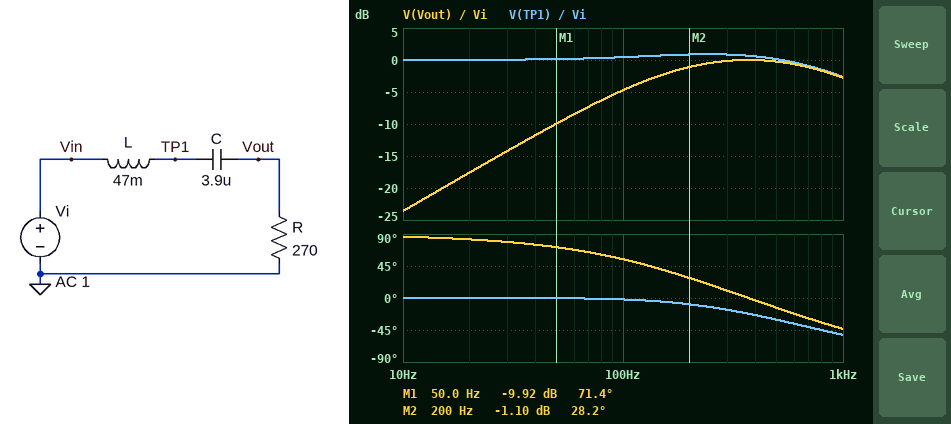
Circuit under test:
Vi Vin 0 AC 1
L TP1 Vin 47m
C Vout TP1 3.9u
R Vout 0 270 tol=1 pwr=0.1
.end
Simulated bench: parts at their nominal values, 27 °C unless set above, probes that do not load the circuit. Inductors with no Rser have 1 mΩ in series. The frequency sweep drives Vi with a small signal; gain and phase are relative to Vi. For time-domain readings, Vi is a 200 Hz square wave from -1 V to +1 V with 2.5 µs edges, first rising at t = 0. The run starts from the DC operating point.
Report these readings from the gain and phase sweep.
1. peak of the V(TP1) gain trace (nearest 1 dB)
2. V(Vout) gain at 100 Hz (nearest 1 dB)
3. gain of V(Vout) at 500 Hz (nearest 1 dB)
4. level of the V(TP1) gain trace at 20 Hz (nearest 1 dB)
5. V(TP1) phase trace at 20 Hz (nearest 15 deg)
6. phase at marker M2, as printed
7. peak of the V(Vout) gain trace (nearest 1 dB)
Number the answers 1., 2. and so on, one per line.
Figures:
1. 1 dB
2. -5 dB
3. 0 dB
4. 0 dB
5. 0 deg
6. 28.2 deg
7. 0 dB
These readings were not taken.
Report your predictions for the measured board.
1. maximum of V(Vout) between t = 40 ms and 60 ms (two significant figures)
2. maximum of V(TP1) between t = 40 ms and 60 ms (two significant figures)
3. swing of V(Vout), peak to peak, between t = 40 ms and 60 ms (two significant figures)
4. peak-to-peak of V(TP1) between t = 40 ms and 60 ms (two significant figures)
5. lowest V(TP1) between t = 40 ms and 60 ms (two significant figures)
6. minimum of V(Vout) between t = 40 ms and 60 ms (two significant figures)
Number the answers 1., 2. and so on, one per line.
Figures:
1. 1.5 V
2. 1.2 V
3. 2.9 V
4. 2.4 V
5. -1.2 V
6. -1.5 V
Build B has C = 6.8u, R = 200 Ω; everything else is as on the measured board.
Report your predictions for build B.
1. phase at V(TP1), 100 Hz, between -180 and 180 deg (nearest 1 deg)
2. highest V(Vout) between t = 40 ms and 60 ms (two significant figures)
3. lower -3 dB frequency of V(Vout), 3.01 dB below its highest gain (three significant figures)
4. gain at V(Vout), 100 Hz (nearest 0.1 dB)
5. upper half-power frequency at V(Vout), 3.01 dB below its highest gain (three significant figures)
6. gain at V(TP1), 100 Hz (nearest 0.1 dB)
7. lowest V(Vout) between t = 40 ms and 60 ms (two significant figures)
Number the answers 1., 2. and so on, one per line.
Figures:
1. -4 deg
2. 1.4 V
3. 102 Hz
4. -3.1 dB
5. 779 Hz
6. 0.6 dB
7. -1.4 V
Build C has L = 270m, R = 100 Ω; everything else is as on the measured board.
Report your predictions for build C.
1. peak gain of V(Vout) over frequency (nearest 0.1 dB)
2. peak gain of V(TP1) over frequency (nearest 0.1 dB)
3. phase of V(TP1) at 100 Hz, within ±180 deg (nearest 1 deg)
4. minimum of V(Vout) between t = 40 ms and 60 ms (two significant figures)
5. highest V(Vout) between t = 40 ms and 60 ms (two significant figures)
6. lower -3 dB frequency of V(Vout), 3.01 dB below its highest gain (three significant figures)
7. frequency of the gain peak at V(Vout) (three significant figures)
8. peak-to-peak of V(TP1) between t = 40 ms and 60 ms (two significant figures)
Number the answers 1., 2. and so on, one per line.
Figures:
1. 0 dB
2. 9.1 dB
3. -9 deg
4. -740 mV
5. 740 mV
6. 128 Hz
7. 155 Hz
8. 3.5 V
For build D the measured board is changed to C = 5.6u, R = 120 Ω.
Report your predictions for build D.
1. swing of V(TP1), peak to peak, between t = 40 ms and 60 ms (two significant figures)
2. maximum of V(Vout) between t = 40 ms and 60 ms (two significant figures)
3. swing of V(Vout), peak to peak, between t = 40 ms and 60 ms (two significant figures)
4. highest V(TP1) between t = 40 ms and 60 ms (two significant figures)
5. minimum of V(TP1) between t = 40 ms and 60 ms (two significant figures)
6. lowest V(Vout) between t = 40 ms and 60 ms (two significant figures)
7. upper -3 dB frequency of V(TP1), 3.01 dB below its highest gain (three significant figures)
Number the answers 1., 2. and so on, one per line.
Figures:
1. 3.0 V
2. 1.3 V
3. 2.6 V
4. 1.5 V
5. -1.5 V
6. -1.3 V
7. 477 Hz
